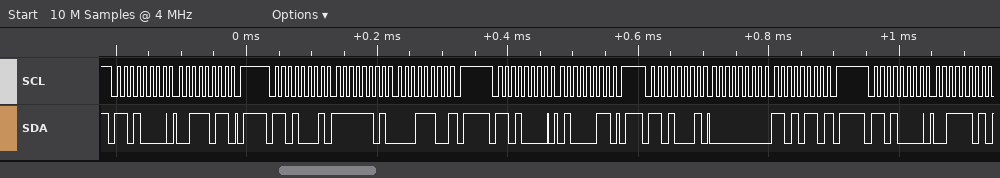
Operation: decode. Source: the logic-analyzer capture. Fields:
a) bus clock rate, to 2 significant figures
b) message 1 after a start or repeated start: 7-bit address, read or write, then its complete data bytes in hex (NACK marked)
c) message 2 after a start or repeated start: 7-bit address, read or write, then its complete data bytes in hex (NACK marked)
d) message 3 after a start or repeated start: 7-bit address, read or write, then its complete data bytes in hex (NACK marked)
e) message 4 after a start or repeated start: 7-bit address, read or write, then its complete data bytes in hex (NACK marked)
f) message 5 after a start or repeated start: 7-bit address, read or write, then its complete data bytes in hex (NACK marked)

100 kHz
0x68 write: 3B
0x68 read: FD 1C NACK
0x68 write: 43
0x68 read: 00 D6 NACK
0x68 write: 3D
